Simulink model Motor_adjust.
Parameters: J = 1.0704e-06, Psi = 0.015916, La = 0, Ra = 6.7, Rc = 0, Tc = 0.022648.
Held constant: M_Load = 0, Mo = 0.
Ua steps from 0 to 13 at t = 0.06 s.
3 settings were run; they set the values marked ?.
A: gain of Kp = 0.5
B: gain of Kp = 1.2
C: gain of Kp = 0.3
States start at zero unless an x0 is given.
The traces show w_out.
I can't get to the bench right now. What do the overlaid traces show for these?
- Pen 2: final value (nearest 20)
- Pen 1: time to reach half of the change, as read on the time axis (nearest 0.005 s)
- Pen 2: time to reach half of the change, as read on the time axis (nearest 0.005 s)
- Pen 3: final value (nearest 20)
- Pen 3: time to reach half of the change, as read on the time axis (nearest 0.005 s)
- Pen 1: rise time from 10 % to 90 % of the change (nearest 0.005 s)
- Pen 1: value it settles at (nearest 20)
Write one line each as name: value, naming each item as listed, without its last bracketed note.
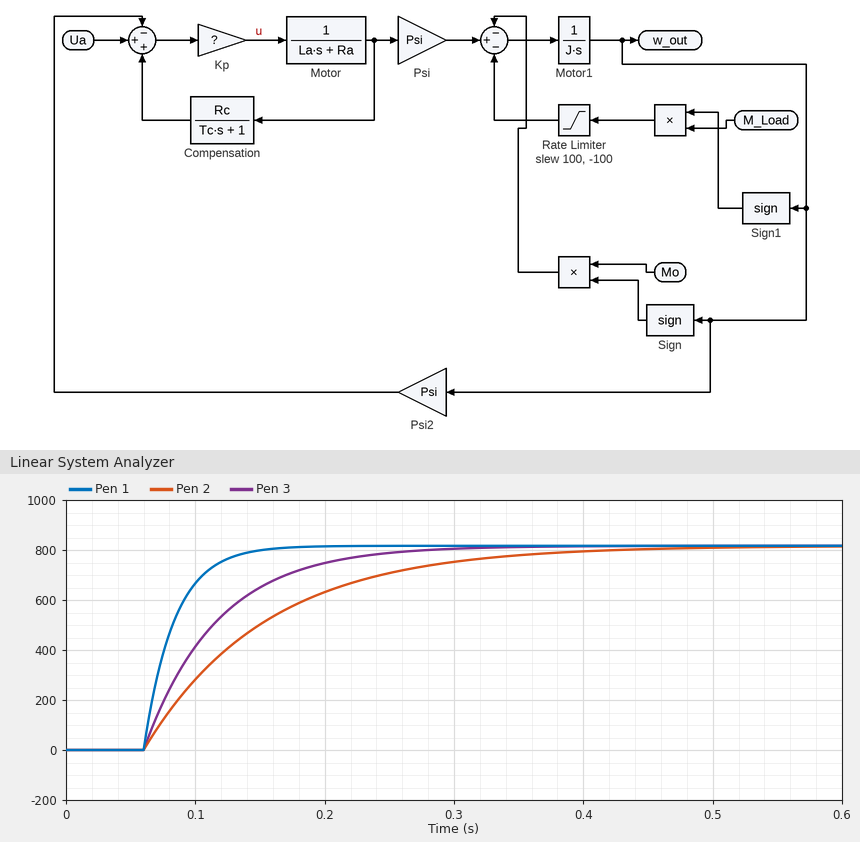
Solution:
Pen 2: final value: 820
Pen 1: time to reach half of the change, as read on the time axis: 0.075 s
Pen 2: time to reach half of the change, as read on the time axis: 0.125 s
Pen 3: final value: 820
Pen 3: time to reach half of the change, as read on the time axis: 0.100 s
Pen 1: rise time from 10 % to 90 % of the change: 0.050 s
Pen 1: value it settles at: 820
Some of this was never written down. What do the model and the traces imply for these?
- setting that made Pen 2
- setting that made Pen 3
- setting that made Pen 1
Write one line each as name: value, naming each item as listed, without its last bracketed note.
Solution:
setting that made Pen 2: C
setting that made Pen 3: A
setting that made Pen 1: B
